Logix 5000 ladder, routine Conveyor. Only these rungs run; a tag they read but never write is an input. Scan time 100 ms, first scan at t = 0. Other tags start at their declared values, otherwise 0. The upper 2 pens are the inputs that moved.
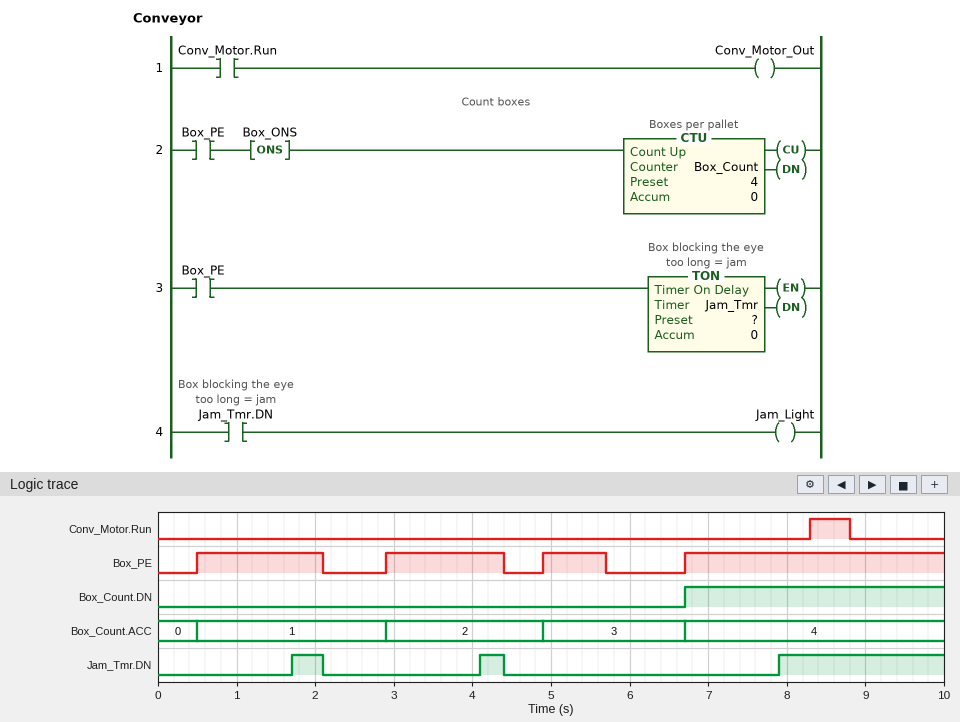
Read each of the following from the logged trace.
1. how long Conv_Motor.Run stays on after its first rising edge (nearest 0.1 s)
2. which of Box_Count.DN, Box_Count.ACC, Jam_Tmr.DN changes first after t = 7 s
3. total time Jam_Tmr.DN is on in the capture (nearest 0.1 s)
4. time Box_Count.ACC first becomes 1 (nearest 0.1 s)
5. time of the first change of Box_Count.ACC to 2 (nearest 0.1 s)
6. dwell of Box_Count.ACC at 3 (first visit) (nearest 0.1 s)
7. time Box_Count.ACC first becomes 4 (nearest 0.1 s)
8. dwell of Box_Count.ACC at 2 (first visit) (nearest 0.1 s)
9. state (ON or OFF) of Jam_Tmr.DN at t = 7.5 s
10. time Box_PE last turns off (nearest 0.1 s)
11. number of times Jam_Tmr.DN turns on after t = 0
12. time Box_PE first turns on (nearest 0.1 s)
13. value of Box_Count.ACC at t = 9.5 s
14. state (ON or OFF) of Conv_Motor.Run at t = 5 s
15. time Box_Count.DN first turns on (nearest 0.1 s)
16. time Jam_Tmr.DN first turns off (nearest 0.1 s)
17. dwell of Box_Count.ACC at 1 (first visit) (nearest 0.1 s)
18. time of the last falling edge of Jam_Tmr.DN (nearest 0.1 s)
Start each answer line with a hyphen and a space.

- 0.5 s
- Jam_Tmr.DN
- 2.8 s
- 0.5 s
- 2.9 s
- 1.8 s
- 6.7 s
- 2.0 s
- OFF
- 5.7 s
- 3
- 0.5 s
- 4
- OFF
- 6.7 s
- 2.1 s
- 2.4 s
- 4.4 s
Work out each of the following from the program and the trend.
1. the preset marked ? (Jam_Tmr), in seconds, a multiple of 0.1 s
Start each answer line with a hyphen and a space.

- 1.2 s
